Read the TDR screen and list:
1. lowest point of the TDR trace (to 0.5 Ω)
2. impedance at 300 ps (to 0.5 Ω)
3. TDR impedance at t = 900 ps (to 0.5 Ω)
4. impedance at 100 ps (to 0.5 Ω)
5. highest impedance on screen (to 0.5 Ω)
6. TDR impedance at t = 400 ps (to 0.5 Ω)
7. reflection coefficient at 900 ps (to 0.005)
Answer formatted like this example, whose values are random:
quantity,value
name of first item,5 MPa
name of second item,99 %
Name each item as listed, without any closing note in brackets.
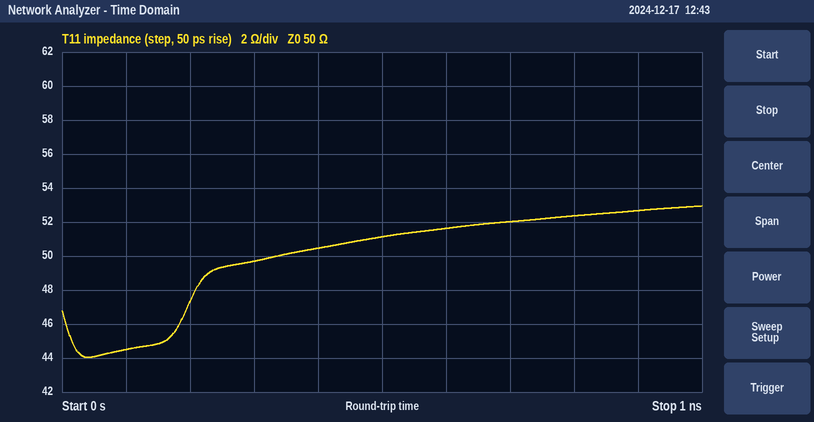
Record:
quantity,value
lowest point of the TDR trace,44.0 Ω
impedance at 300 ps,49.5 Ω
TDR impedance at t = 900 ps,52.5 Ω
impedance at 100 ps,44.5 Ω
highest impedance on screen,53.0 Ω
TDR impedance at t = 400 ps,50.5 Ω
reflection coefficient at 900 ps,+0.025
